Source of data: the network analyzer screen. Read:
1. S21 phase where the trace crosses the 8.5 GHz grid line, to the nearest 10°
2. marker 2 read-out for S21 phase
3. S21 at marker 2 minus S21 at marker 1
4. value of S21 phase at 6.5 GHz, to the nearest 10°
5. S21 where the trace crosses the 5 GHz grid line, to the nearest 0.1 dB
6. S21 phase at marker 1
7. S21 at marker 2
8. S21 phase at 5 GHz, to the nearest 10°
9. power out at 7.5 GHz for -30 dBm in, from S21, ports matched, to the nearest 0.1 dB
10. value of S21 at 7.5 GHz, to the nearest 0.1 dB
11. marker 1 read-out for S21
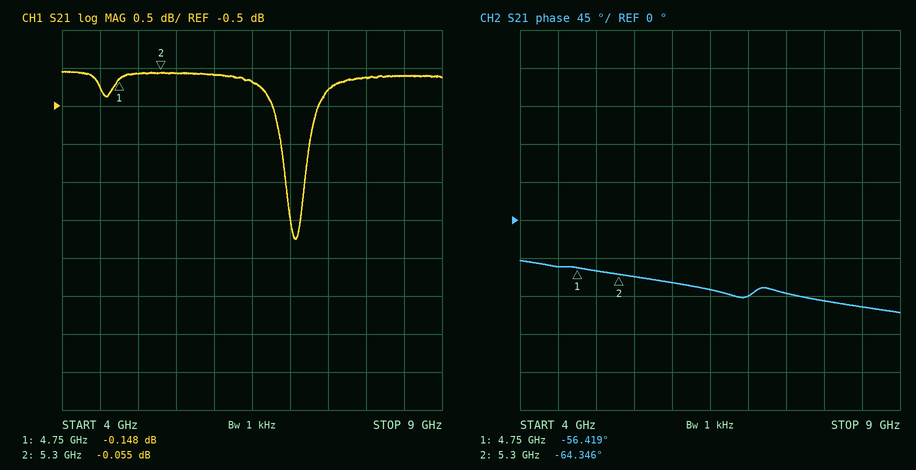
-100°
-64.346°
0.093 dB
-80°
-0.1 dB
-56.419°
-0.055 dB
-60°
-30.3 dBm
-0.3 dB
-0.148 dB
